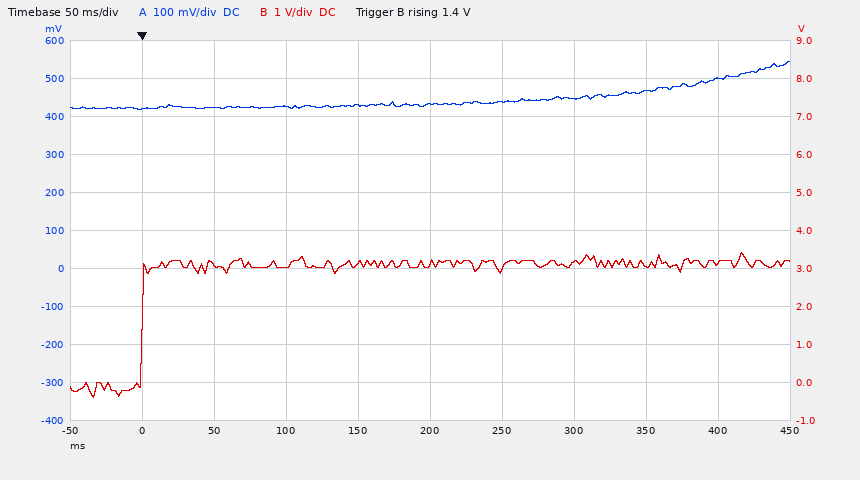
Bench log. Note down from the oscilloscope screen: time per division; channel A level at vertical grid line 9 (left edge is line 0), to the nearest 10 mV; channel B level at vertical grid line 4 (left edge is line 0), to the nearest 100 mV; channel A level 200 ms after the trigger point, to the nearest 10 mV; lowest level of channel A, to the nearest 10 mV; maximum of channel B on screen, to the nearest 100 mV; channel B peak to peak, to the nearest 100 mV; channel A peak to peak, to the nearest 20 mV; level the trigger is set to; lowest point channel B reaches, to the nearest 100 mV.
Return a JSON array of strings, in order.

["50 ms", "500 mV", "3.1 V", "430 mV", "420 mV", "3.4 V", "3.8 V", "120 mV", "1.4 V", "-400 mV"]
